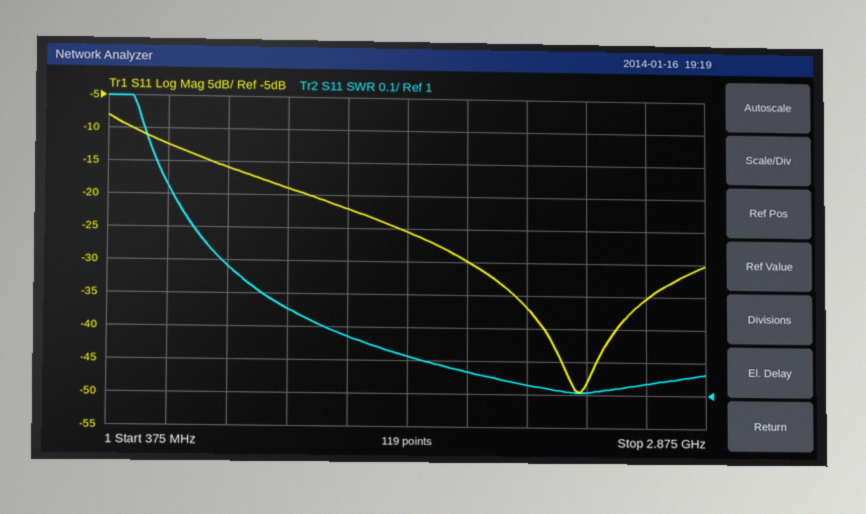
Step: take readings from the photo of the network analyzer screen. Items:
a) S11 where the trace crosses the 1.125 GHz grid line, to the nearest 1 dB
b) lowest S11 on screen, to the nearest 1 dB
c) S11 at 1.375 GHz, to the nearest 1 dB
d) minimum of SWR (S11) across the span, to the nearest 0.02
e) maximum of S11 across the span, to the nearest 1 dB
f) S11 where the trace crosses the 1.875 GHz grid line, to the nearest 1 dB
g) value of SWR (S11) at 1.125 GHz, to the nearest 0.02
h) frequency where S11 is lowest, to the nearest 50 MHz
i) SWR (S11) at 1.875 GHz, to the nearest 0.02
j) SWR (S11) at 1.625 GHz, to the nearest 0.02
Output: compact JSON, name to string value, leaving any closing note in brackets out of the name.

{"S11 where the trace crosses the 1.125 GHz grid line, to the nearest 1 dB": "-19 dB", "lowest S11 on screen, to the nearest 1 dB": "-50 dB", "S11 at 1.375 GHz, to the nearest 1 dB": "-22 dB", "minimum of SWR (S11) across the span, to the nearest 0.02": "1.00", "maximum of S11 across the span, to the nearest 1 dB": "-8 dB", "S11 where the trace crosses the 1.875 GHz grid line, to the nearest 1 dB": "-30 dB", "value of SWR (S11) at 1.125 GHz, to the nearest 0.02": "1.26", "frequency where S11 is lowest, to the nearest 50 MHz": "2.35 GHz", "SWR (S11) at 1.875 GHz, to the nearest 0.02": "1.06", "SWR (S11) at 1.625 GHz, to the nearest 0.02": "1.12"}
